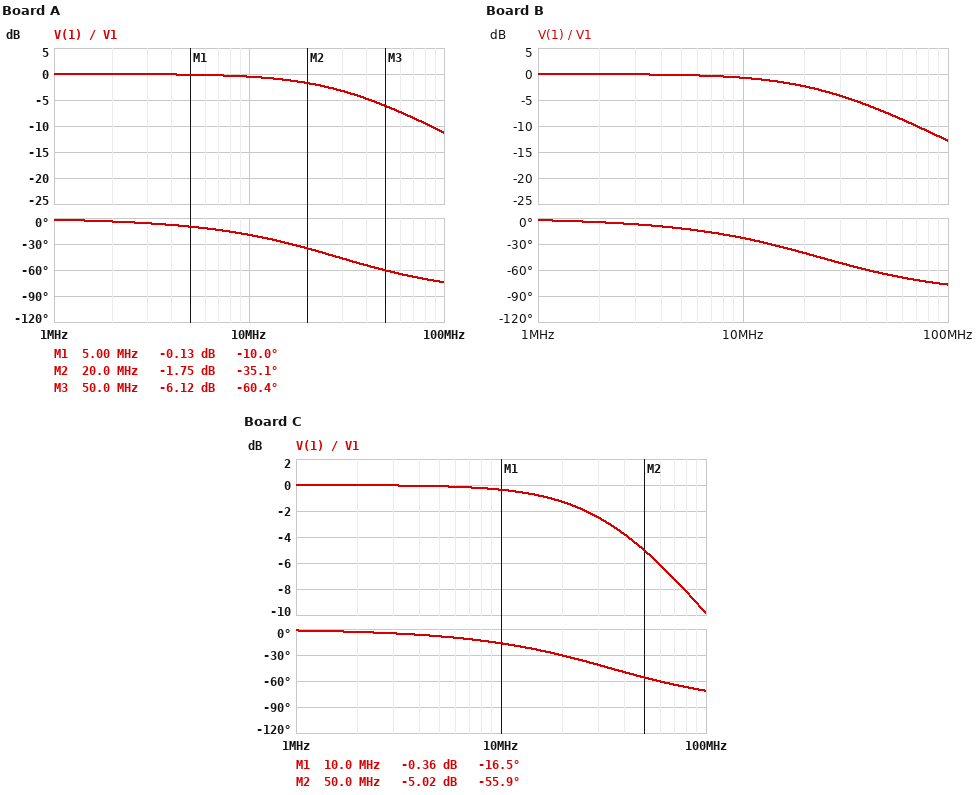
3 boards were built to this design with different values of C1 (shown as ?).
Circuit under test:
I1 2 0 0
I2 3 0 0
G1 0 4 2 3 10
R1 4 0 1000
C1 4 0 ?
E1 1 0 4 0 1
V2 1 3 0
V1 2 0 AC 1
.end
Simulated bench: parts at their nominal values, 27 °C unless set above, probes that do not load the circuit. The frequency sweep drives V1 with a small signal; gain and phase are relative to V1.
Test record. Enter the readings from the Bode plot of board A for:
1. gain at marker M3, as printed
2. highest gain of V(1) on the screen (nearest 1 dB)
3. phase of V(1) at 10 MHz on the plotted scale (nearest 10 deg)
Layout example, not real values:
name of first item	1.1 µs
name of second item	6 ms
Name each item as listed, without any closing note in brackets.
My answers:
gain at marker M3, as printed	-6.12 dB
highest gain of V(1) on the screen	0 dB
phase of V(1) at 10 MHz on the plotted scale	-20 deg
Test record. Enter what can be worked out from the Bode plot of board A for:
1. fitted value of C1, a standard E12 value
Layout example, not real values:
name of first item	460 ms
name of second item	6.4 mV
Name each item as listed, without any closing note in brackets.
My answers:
fitted value of C1, a standard E12 value	56 nF
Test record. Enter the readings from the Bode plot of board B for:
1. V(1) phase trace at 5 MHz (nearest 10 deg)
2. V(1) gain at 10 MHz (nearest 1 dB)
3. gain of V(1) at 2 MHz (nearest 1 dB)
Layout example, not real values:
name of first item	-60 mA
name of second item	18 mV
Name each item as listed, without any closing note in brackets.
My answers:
V(1) phase trace at 5 MHz	-10 deg
V(1) gain at 10 MHz	-1 dB
gain of V(1) at 2 MHz	0 dB
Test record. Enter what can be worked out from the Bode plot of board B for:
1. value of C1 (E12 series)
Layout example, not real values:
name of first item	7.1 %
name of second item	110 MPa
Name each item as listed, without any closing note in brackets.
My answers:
value of C1	68 nF
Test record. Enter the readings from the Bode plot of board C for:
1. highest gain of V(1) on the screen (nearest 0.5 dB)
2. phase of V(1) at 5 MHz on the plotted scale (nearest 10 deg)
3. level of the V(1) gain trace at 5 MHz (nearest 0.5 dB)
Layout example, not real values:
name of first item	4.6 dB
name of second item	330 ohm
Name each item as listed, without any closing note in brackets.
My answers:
highest gain of V(1) on the screen	0 dB
phase of V(1) at 5 MHz on the plotted scale	-10 deg
level of the V(1) gain trace at 5 MHz	0 dB
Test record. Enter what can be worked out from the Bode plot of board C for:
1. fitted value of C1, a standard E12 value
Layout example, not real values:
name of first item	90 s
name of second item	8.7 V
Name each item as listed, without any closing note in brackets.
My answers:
fitted value of C1, a standard E12 value	47 nF
